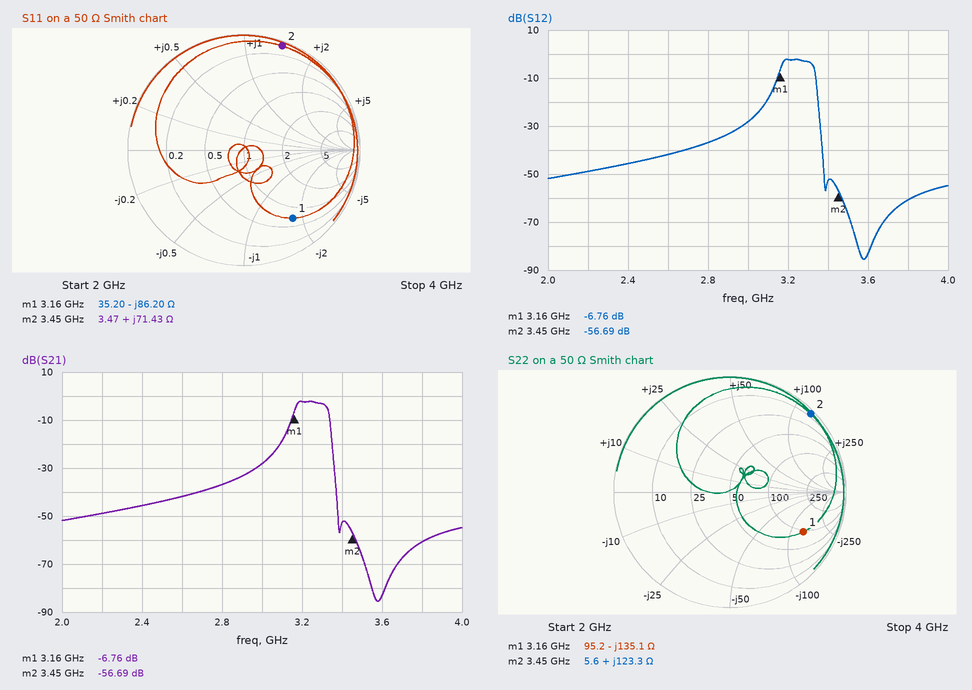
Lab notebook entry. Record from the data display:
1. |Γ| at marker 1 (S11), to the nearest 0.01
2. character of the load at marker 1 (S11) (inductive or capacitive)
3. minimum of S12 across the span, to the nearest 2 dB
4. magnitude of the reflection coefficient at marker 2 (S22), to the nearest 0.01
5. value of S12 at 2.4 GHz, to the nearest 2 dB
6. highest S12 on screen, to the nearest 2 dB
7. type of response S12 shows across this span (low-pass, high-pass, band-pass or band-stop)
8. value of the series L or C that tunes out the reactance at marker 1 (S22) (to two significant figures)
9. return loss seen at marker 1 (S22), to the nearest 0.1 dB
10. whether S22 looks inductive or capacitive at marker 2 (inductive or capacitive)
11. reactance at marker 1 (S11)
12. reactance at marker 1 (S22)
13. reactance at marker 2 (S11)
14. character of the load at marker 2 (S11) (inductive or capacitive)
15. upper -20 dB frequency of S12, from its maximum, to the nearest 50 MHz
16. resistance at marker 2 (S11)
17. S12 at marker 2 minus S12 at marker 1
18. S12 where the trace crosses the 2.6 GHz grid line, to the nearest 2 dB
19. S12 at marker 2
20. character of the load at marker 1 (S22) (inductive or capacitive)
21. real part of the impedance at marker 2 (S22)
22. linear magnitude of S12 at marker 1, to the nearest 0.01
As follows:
0.72
capacitive
-86 dB
0.97
-46 dB
-2 dB
band-pass
6.8 nH
2.9 dB
inductive
-86.20 Ω
-135.1 Ω
+71.43 Ω
inductive
3.35 GHz
3.47 Ω
-49.93 dB
-42 dB
-56.69 dB
capacitive
5.6 Ω
0.46
